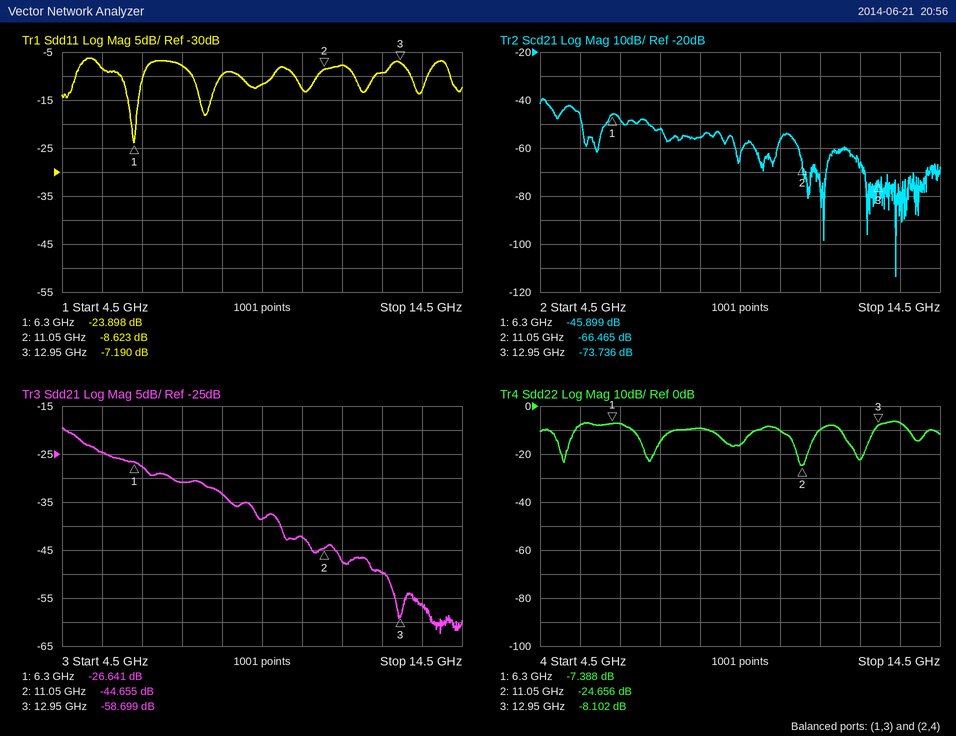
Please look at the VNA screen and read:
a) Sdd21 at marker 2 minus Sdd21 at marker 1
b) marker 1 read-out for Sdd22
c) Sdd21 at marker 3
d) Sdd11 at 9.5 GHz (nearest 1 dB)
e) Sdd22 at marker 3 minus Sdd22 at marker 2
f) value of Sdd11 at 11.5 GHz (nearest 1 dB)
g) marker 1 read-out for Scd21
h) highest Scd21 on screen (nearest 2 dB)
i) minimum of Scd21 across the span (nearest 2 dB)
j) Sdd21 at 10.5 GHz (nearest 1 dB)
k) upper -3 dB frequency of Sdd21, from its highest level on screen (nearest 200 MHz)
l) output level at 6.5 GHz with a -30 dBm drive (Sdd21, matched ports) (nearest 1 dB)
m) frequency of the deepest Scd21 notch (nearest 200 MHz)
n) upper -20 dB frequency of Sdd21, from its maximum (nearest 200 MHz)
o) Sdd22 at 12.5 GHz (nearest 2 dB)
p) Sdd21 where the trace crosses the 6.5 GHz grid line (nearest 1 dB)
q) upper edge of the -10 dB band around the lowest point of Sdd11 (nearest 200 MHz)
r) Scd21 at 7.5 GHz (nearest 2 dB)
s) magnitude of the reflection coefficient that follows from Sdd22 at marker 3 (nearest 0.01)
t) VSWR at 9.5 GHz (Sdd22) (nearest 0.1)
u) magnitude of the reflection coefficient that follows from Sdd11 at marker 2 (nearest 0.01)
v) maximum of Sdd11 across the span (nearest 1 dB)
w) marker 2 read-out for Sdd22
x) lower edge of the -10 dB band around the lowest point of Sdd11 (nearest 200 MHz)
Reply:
-18.014 dB
-7.388 dB
-58.699 dB
-12 dB
16.554 dB
-8 dB
-45.899 dB
-40 dB
-114 dB
-42 dB
5.0 GHz
-58 dBm
13.4 GHz
10.0 GHz
-22 dB
-28 dB
6.6 GHz
-52 dB
0.39
1.4
0.37
-6 dB
-24.656 dB
6.0 GHz
